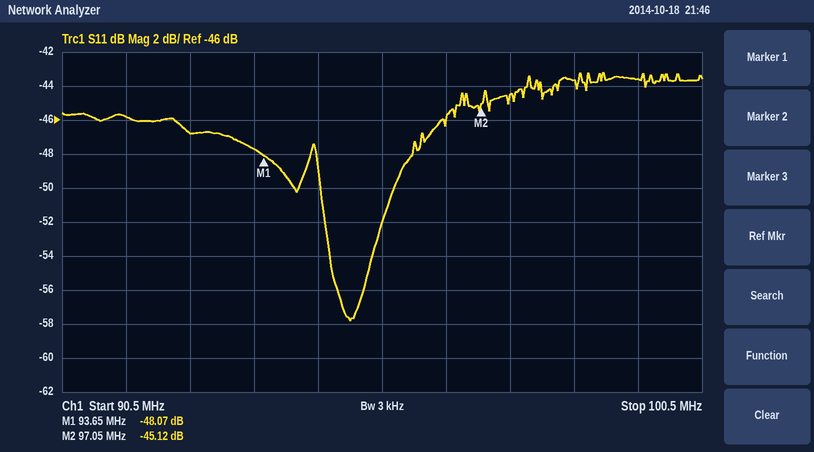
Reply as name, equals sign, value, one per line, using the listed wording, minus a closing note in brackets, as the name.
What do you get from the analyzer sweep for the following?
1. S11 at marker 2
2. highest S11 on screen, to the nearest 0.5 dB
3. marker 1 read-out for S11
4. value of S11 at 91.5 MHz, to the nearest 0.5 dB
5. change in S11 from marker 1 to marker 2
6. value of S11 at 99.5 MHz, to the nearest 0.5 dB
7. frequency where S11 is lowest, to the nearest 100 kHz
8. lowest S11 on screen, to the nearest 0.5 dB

S11 at marker 2 = -45.12 dB
highest S11 on screen, to the nearest 0.5 dB = -43.0 dB
marker 1 read-out for S11 = -48.07 dB
value of S11 at 91.5 MHz, to the nearest 0.5 dB = -46.0 dB
change in S11 from marker 1 to marker 2 = 2.95 dB
value of S11 at 99.5 MHz, to the nearest 0.5 dB = -43.5 dB
frequency where S11 is lowest, to the nearest 100 kHz = 95.0 MHz
lowest S11 on screen, to the nearest 0.5 dB = -58.0 dB
